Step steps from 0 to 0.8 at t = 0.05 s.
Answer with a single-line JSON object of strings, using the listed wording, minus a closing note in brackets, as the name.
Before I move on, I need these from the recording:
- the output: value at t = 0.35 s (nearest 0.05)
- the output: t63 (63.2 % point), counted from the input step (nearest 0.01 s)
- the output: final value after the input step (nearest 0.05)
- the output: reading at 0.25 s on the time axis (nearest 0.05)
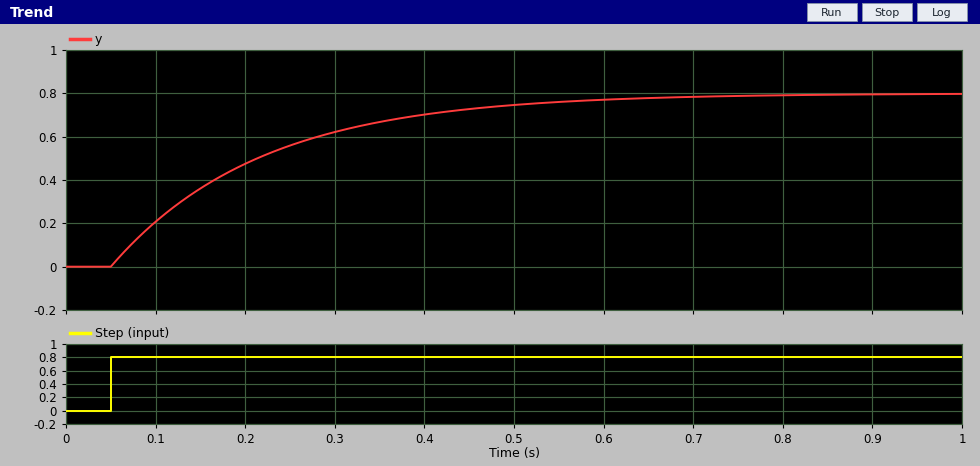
{"the output: value at t = 0.35 s": "0.65", "the output: t63 (63.2 % point), counted from the input step": "0.17 s", "the output: final value after the input step": "0.80", "the output: reading at 0.25 s on the time axis": "0.55"}
